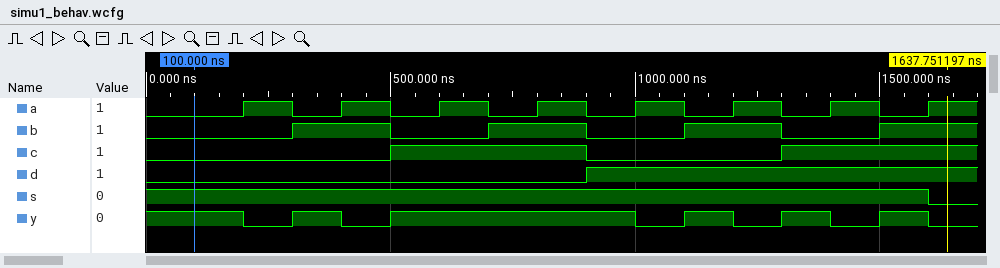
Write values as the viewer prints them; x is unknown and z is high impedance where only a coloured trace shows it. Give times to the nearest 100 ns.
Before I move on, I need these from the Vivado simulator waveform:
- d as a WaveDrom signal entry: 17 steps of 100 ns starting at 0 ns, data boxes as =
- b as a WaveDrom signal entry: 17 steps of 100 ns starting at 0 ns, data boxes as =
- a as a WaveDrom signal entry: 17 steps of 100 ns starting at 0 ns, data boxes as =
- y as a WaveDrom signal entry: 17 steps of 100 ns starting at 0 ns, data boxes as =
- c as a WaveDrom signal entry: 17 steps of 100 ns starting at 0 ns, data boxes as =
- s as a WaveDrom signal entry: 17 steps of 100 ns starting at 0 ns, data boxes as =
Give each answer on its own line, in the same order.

{name: 'd', wave: '0........1.......'}
{name: 'b', wave: '0..1.0.1.0.1.0.1.'}
{name: 'a', wave: '0.101010101010101'}
{name: 'y', wave: '1.0101....0101010'}
{name: 'c', wave: '0....1...0...1...'}
{name: 's', wave: '1...............0'}
